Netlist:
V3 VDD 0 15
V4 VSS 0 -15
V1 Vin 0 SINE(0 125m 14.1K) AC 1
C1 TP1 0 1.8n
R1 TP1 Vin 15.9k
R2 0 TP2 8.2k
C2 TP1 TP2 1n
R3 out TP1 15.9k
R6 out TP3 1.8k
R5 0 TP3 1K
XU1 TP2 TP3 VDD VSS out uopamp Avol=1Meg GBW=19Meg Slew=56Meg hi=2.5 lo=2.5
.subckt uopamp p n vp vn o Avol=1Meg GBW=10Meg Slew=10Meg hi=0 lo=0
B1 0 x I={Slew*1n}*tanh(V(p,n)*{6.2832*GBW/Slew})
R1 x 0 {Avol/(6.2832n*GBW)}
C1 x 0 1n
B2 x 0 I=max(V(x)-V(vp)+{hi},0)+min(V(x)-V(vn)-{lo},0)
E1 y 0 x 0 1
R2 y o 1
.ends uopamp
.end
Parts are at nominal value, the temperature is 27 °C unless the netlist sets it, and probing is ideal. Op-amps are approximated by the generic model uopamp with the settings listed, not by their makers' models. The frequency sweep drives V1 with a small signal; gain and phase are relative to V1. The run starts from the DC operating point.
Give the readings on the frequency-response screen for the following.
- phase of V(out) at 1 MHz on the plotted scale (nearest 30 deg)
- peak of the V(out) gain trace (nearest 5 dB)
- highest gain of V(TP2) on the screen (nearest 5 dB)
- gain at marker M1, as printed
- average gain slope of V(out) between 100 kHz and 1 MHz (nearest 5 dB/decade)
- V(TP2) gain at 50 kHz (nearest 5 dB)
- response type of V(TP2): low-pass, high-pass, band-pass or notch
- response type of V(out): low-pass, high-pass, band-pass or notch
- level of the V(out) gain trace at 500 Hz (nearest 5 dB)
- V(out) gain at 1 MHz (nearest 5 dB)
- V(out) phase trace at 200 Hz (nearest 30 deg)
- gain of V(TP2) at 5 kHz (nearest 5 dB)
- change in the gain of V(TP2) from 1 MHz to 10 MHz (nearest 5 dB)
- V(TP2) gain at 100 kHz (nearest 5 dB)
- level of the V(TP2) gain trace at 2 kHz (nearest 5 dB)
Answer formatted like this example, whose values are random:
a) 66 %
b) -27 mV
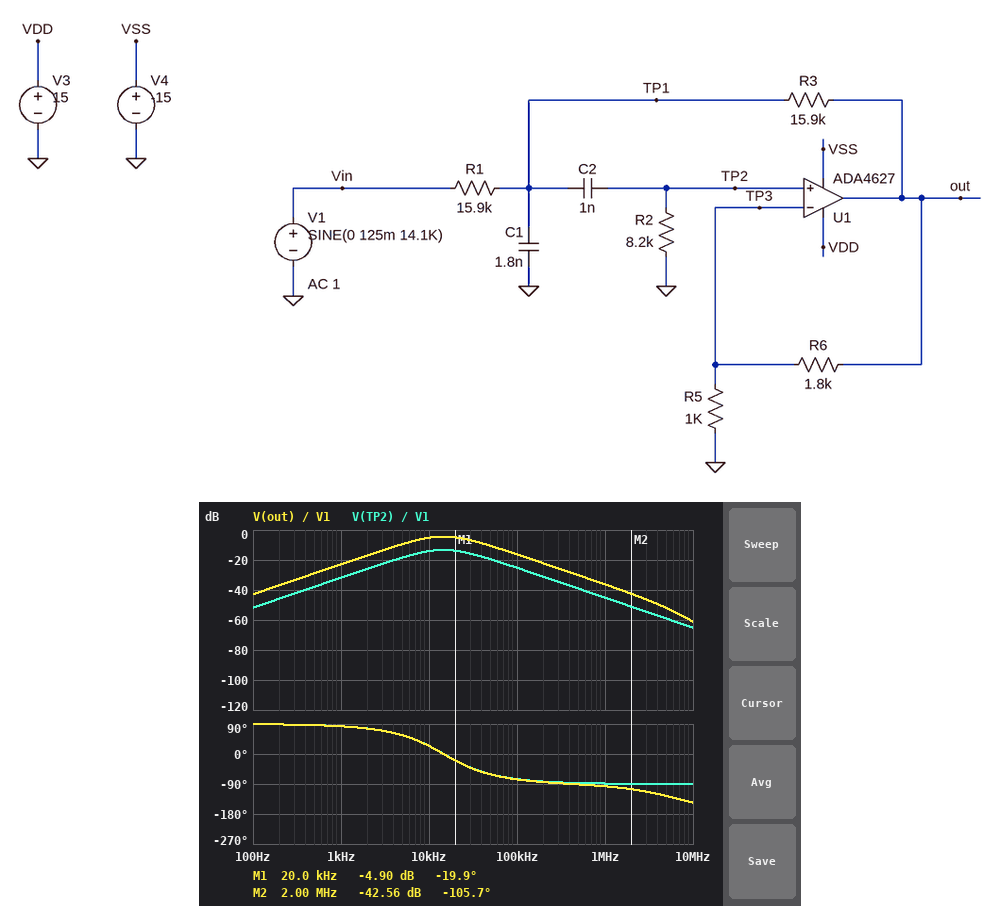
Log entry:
a) -90 deg
b) -5 dB
c) -15 dB
d) -4.90 dB
e) -20 dB/decade
f) -20 dB
g) band-pass
h) band-pass
i) -30 dB
j) -35 dB
k) 90 deg
l) -20 dB
m) -20 dB
n) -25 dB
o) -25 dB
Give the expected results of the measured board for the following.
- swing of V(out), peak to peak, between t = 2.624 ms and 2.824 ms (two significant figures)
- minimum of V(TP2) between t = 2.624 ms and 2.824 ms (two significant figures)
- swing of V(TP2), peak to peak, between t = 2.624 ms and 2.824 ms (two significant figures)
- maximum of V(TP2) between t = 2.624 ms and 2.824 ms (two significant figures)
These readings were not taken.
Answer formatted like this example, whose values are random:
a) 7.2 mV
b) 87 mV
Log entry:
a) 150 mV
b) -27 mV
c) 54 mV
d) 27 mV
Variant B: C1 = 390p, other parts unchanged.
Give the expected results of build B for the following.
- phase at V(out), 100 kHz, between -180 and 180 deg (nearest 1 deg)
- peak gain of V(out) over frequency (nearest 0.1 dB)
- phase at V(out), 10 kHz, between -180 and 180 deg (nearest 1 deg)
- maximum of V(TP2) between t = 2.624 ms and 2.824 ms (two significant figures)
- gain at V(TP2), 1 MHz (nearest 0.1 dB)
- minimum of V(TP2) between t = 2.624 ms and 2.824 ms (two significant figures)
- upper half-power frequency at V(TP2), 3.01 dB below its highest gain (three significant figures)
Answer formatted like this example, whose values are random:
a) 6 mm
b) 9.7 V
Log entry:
a) -63 deg
b) 3.4 dB
c) 61 deg
d) 43 mV
e) -31.9 dB
f) -43 mV
g) 63.6 kHz
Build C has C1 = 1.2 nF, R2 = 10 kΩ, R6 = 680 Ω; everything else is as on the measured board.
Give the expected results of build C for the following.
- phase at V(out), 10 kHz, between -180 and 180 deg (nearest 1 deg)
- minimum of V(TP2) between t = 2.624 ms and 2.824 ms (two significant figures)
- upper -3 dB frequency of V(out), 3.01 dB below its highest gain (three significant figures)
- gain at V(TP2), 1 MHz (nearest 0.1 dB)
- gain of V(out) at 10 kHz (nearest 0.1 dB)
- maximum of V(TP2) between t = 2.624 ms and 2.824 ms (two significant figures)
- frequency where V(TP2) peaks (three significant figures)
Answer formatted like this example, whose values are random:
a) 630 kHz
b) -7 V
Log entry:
a) 27 deg
b) -32 mV
c) 38.7 kHz
d) -41.6 dB
e) -8.2 dB
f) 32 mV
g) 16.3 kHz
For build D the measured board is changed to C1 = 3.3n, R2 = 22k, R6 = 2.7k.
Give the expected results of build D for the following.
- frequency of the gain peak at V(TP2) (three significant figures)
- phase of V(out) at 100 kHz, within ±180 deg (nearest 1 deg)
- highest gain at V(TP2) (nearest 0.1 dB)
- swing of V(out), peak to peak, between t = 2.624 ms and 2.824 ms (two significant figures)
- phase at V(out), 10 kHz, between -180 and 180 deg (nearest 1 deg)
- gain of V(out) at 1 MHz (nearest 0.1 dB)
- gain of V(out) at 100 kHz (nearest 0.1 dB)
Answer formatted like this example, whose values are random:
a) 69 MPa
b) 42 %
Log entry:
a) 6.62 kHz
b) -89 deg
c) -3.0 dB
d) 240 mV
e) -53 deg
f) -39.2 dB
g) -19.0 dB
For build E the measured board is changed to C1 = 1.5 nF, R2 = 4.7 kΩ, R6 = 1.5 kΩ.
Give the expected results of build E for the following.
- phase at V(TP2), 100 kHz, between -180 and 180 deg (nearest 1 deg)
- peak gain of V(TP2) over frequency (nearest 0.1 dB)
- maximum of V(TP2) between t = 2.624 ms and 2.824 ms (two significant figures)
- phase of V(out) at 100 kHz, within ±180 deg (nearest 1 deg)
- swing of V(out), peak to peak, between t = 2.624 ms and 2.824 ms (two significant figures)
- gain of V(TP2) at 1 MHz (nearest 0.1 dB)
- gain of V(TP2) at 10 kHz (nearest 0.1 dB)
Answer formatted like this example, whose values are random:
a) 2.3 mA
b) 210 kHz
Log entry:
a) -61 deg
b) -18.0 dB
c) 15 mV
d) -62 deg
e) 74 mV
f) -43.5 dB
g) -19.6 dB
